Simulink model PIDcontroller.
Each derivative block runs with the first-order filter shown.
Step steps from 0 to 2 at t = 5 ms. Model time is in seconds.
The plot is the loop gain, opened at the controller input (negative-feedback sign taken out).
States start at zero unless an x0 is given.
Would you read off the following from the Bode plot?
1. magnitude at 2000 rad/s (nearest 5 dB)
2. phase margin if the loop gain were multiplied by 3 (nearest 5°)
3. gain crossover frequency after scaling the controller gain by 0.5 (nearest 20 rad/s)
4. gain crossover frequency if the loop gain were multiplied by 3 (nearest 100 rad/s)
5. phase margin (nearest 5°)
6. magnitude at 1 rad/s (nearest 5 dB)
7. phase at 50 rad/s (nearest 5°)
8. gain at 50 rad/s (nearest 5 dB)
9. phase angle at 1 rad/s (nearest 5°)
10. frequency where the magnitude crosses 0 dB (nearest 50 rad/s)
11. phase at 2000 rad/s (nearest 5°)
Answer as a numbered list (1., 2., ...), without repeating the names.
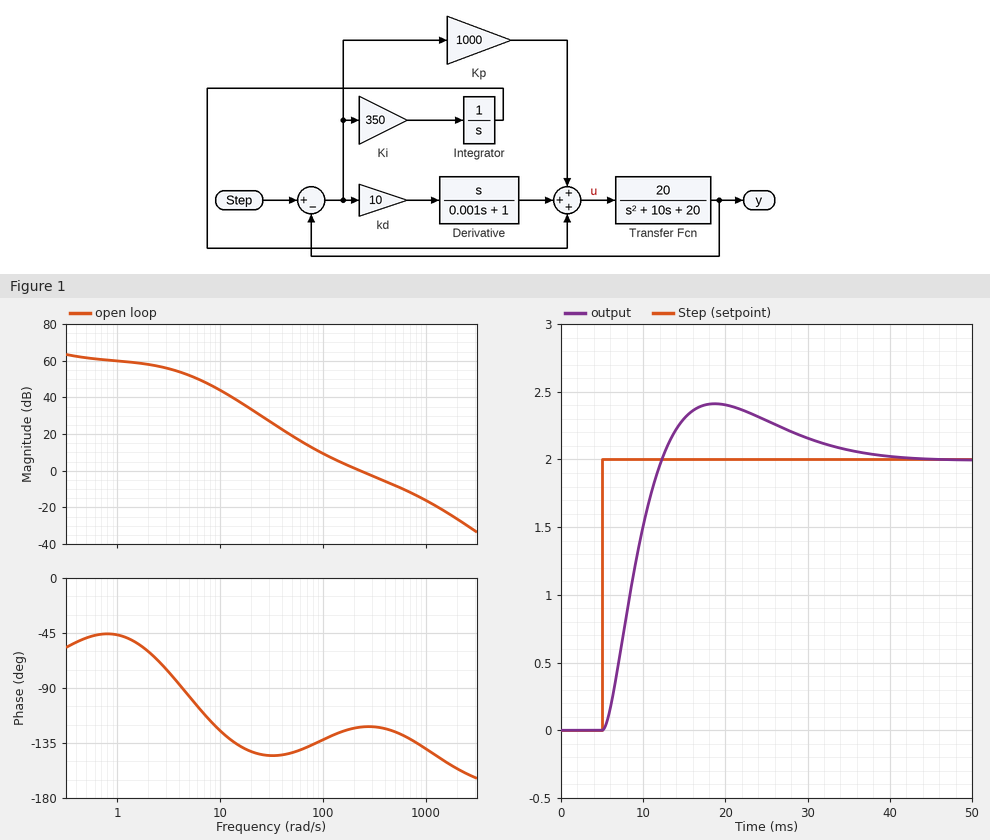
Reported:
1. -25 dB
2. 50°
3. 140 rad/s
4. 600 rad/s
5. 60°
6. 60 dB
7. -145°
8. 20 dB
9. -45°
10. 250 rad/s
11. -155°
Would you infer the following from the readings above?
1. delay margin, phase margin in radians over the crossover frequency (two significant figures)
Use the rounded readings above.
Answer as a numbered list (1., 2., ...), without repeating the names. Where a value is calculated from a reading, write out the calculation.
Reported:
1. 60 × π / 180 / 250 = 0.0042 s
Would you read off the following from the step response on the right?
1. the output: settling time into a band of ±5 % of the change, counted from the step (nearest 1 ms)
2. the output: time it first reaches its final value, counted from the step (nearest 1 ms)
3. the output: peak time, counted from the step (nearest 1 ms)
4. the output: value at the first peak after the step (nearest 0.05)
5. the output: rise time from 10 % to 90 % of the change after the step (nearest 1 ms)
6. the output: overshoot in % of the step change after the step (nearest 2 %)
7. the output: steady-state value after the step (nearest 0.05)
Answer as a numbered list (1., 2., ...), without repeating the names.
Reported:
1. 28 ms
2. 7 ms
3. 14 ms
4. 2.40
5. 5 ms
6. 20 %
7. 2.00
